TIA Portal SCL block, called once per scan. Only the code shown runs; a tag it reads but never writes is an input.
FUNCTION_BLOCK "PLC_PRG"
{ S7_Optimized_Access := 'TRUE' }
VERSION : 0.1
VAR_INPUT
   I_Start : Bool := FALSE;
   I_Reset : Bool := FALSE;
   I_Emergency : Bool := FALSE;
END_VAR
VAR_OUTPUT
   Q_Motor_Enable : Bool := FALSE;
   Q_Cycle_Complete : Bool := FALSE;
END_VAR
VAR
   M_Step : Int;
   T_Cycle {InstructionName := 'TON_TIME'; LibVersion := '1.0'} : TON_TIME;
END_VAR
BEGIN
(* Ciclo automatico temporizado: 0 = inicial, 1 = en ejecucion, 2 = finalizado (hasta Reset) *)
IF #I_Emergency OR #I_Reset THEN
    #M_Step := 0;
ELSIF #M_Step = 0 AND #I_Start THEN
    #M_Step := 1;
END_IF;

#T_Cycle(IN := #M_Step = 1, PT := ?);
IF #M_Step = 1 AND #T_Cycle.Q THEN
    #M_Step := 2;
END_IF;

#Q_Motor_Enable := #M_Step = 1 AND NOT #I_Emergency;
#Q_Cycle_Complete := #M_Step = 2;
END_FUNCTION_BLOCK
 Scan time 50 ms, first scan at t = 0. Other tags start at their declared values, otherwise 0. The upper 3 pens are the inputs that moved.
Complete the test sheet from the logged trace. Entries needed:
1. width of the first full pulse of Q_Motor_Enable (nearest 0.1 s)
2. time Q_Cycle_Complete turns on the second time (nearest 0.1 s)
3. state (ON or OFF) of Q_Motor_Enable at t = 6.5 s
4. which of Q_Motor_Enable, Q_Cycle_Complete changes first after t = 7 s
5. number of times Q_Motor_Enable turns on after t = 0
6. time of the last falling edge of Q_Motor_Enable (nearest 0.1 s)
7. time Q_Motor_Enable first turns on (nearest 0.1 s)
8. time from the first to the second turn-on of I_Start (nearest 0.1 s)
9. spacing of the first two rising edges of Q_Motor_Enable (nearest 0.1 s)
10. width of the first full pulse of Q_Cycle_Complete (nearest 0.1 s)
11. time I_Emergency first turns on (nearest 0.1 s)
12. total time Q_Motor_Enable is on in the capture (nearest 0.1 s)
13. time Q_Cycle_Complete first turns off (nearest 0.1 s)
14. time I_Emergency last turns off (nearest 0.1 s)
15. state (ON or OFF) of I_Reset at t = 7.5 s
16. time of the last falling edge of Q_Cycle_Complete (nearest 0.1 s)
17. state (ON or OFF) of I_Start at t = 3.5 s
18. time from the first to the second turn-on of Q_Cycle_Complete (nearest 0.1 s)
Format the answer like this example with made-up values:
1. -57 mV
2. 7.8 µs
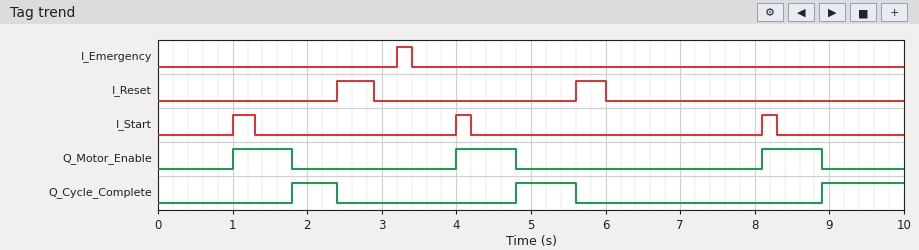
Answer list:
1. 0.8 s
2. 4.8 s
3. OFF
4. Q_Motor_Enable
5. 3
6. 8.9 s
7. 1.0 s
8. 3.0 s
9. 3.0 s
10. 0.6 s
11. 3.2 s
12. 2.4 s
13. 2.4 s
14. 3.4 s
15. OFF
16. 5.6 s
17. OFF
18. 3.0 s
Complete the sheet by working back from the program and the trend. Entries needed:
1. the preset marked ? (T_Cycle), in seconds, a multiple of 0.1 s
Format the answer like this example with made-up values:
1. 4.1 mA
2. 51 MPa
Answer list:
1. 0.8 s
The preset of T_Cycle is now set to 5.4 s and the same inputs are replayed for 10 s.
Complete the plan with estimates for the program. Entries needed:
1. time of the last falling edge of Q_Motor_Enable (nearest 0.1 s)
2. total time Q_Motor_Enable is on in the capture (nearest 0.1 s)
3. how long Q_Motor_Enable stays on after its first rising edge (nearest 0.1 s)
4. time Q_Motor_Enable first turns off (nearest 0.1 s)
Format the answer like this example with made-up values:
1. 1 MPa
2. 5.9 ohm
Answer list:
1. 5.6 s
2. 4.9 s
3. 1.4 s
4. 2.4 s
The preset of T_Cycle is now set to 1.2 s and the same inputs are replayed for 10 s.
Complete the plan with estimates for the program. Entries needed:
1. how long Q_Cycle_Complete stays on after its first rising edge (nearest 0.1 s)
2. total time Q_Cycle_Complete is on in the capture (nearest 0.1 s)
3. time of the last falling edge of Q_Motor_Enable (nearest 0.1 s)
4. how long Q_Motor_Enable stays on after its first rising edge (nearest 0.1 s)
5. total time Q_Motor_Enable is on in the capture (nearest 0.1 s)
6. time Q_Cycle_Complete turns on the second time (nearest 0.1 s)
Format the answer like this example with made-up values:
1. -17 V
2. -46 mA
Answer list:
1. 0.2 s
2. 1.3 s
3. 9.3 s
4. 1.2 s
5. 3.6 s
6. 5.2 s
